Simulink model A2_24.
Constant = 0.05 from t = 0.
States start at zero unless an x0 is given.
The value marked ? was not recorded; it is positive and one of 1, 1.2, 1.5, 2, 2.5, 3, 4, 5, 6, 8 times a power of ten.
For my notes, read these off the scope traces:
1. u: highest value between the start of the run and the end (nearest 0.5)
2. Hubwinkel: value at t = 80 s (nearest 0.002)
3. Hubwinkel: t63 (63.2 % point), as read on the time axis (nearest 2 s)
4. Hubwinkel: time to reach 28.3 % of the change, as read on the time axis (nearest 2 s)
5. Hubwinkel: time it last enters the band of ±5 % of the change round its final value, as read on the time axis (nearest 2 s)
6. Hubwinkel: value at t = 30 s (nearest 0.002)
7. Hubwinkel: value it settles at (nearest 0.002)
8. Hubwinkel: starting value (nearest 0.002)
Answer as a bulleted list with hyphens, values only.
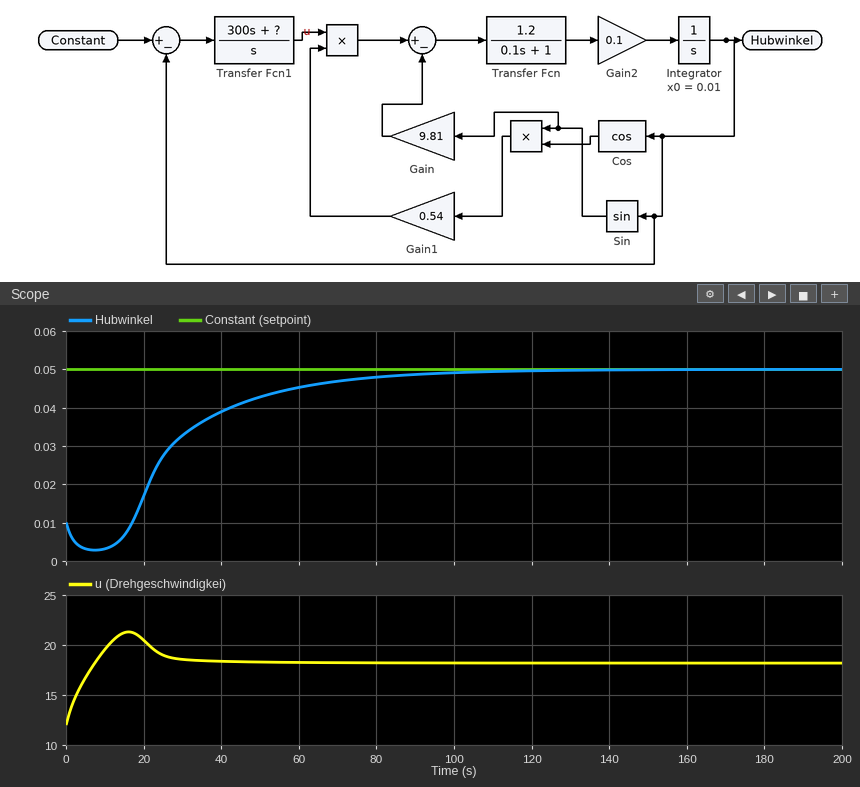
- 21.5
- 0.048
- 34 s
- 22 s
- 80 s
- 0.032
- 0.050
- 0.010
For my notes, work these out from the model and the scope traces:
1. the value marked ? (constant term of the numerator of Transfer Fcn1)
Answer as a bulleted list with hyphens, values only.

- 12
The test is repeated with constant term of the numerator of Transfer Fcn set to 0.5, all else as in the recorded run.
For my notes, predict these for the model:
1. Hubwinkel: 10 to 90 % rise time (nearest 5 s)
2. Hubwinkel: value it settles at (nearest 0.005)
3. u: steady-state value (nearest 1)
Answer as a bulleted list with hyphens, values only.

- 35 s
- 0.050
- 18
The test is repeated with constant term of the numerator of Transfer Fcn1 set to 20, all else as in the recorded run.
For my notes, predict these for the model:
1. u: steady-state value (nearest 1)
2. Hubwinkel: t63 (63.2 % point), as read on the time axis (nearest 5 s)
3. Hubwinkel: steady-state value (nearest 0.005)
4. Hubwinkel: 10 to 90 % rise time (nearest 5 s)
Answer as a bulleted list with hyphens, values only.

- 18
- 20 s
- 0.050
- 25 s
